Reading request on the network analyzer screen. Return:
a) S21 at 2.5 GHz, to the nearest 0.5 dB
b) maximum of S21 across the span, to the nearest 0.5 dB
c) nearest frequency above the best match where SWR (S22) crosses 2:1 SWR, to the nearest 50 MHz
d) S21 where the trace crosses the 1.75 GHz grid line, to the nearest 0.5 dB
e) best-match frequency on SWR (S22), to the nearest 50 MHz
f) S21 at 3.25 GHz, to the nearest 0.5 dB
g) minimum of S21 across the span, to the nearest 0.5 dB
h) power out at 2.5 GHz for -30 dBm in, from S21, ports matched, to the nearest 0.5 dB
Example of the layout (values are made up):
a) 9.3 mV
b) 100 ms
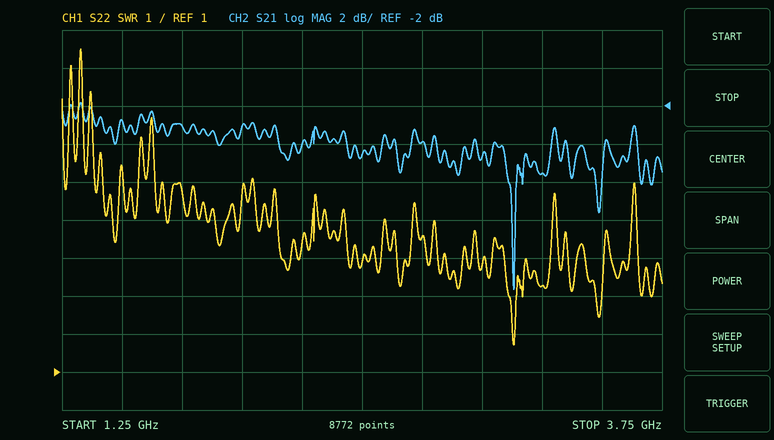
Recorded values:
a) -4.5 dB
b) -2.0 dB
c) 3.15 GHz
d) -3.0 dB
e) 3.15 GHz
f) -5.5 dB
g) -11.5 dB
h) -34.5 dBm
